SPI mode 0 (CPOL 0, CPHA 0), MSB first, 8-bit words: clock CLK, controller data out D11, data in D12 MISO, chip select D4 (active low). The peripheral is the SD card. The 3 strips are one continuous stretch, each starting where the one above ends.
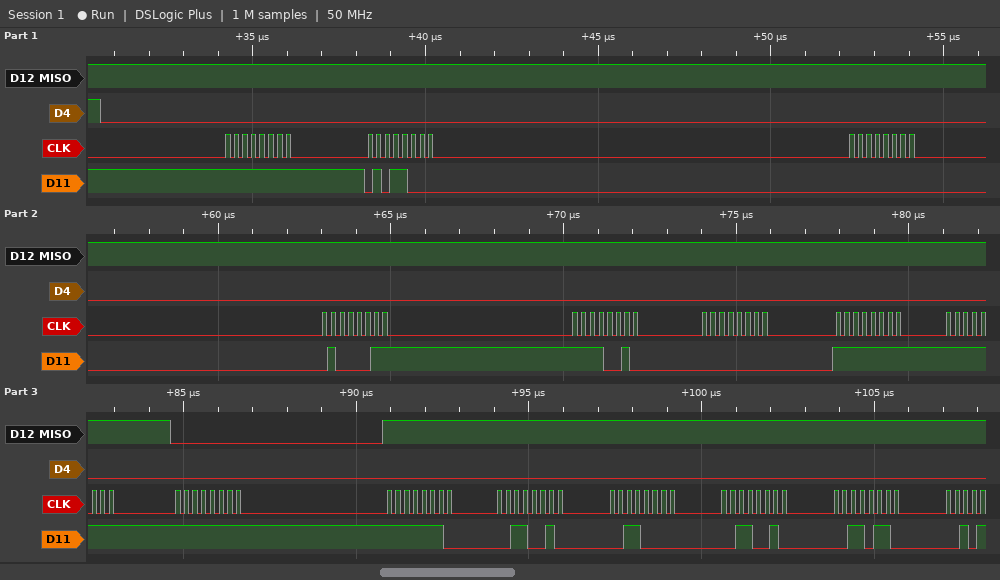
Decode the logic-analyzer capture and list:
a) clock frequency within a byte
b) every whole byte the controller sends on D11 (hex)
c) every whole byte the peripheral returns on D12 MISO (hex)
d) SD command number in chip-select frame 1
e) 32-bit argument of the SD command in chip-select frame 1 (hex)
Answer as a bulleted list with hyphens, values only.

- 4 MHz
- FF 58 00 43 F2 00 FF FF FF FE 32 30 32 36
- FF FF FF FF FF FF FF FF 00 FF FF FF FF FF
- CMD24
- 0x0043F200
